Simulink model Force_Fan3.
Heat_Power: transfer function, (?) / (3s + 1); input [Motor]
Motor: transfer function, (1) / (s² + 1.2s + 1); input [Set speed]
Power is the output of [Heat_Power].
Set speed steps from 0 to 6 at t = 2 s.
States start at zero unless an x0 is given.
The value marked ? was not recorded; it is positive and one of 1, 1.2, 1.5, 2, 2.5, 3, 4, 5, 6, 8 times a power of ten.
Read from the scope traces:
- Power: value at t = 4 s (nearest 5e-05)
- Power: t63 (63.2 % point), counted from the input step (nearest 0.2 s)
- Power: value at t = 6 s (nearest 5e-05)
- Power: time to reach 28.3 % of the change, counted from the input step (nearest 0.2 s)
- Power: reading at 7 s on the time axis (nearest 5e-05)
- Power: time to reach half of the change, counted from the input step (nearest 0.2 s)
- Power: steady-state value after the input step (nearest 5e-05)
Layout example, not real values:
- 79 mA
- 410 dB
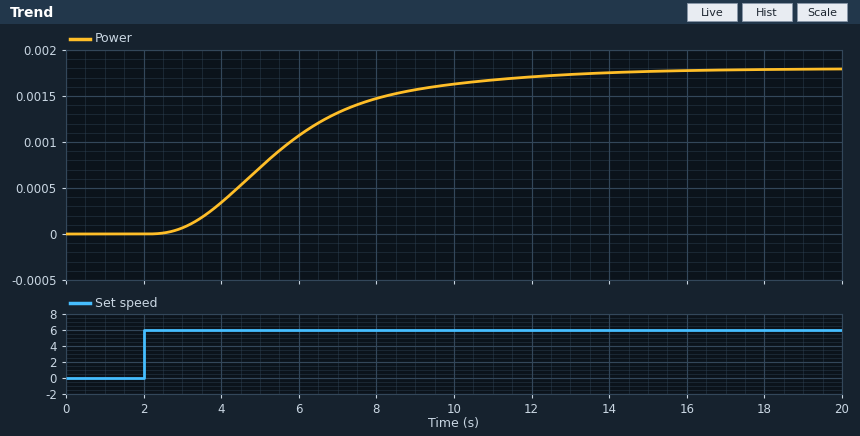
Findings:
- 0.00035
- 4.2 s
- 0.00105
- 2.4 s
- 0.00130
- 3.4 s
- 0.00180
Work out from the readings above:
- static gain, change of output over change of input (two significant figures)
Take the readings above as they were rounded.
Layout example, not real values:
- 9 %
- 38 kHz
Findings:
- 0.00030
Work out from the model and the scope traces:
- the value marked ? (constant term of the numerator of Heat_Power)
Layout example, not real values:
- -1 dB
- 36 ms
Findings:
- 0.0003
